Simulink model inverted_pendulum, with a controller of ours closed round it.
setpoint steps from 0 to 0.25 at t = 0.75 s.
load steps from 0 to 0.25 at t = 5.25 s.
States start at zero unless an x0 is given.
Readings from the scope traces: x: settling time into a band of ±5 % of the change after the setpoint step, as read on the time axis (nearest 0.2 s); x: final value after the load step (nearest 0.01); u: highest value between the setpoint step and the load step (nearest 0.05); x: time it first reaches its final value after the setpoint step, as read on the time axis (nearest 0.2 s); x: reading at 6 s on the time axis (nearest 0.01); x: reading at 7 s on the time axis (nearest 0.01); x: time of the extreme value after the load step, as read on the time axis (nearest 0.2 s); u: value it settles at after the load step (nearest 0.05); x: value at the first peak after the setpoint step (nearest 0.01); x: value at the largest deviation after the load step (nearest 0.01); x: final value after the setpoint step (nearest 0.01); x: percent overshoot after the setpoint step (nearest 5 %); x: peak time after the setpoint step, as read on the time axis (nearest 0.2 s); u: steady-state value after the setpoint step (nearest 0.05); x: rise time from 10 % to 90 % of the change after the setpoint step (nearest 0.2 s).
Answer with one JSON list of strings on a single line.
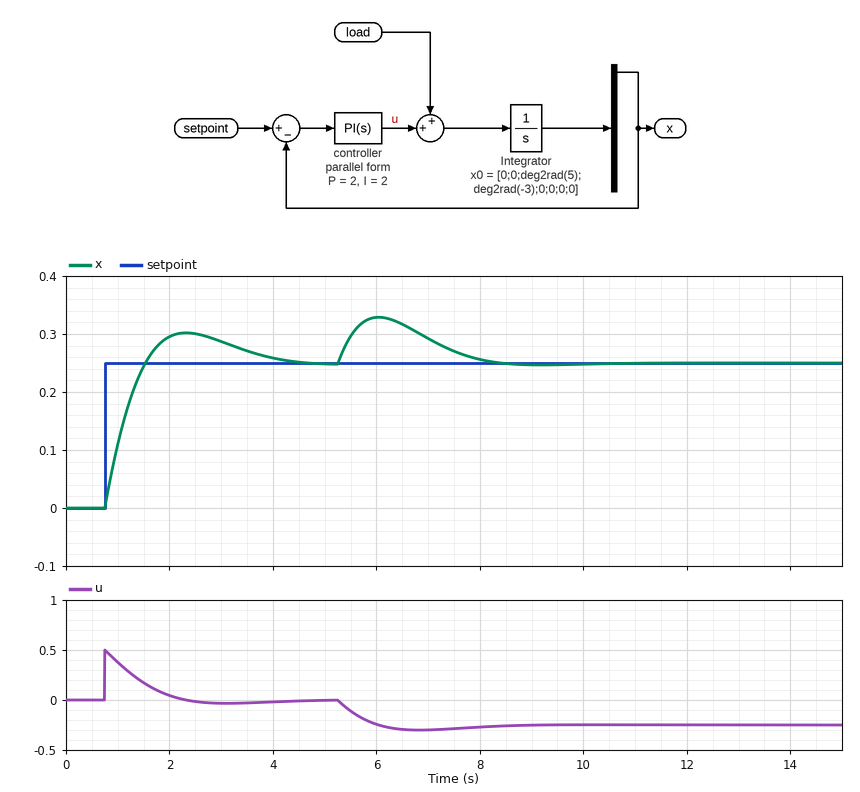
["3.8 s", "0.25", "0.50", "1.6 s", "0.33", "0.29", "6.0 s", "-0.25", "0.30", "0.33", "0.25", "20 %", "2.4 s", "0.00", "0.6 s"]
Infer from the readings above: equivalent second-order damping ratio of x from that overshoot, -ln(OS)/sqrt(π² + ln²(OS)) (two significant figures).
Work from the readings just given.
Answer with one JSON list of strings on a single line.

["0.46"]
